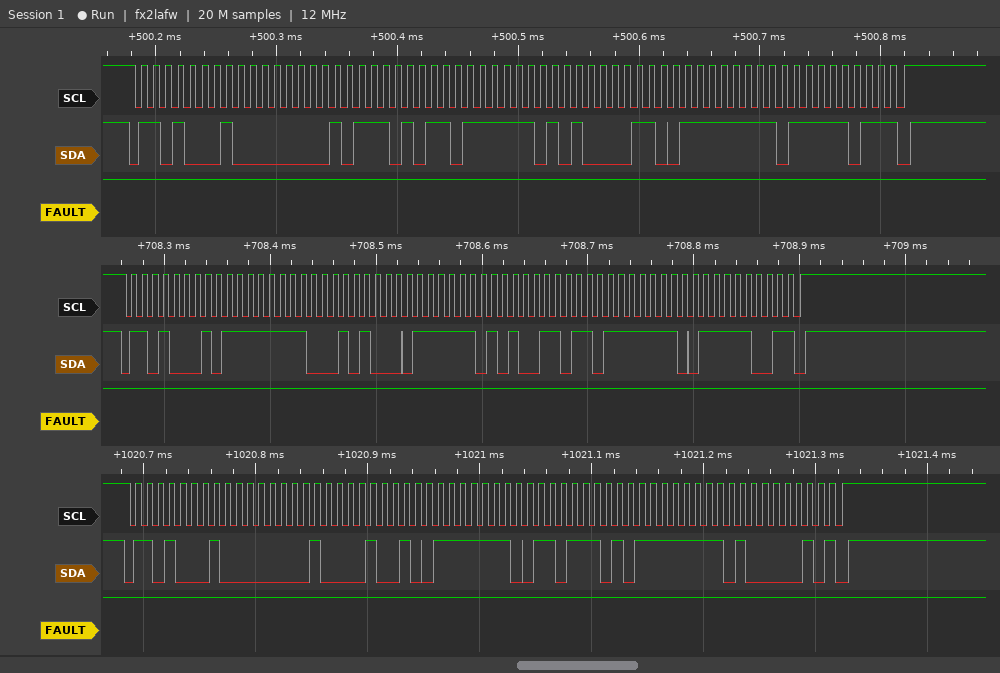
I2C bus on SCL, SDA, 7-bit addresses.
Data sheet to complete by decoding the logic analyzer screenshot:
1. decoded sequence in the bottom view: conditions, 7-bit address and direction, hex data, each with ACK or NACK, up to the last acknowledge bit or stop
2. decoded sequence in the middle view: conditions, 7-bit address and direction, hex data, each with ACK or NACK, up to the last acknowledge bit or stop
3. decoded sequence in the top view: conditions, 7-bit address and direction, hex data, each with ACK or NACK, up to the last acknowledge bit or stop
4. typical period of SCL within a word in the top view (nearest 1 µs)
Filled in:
start, address 68 read ACK, 01 ACK, 12 ACK, FE ACK, DD ACK, FF ACK, 82 NACK, stop
start, address 68 read ACK, FF ACK, 28 ACK, FD ACK, 9B ACK, FE ACK, F9 NACK, stop
start, address 68 read ACK, 01 ACK, EB ACK, FD ACK, 86 ACK, FF ACK, FB NACK, stop
10 µs
